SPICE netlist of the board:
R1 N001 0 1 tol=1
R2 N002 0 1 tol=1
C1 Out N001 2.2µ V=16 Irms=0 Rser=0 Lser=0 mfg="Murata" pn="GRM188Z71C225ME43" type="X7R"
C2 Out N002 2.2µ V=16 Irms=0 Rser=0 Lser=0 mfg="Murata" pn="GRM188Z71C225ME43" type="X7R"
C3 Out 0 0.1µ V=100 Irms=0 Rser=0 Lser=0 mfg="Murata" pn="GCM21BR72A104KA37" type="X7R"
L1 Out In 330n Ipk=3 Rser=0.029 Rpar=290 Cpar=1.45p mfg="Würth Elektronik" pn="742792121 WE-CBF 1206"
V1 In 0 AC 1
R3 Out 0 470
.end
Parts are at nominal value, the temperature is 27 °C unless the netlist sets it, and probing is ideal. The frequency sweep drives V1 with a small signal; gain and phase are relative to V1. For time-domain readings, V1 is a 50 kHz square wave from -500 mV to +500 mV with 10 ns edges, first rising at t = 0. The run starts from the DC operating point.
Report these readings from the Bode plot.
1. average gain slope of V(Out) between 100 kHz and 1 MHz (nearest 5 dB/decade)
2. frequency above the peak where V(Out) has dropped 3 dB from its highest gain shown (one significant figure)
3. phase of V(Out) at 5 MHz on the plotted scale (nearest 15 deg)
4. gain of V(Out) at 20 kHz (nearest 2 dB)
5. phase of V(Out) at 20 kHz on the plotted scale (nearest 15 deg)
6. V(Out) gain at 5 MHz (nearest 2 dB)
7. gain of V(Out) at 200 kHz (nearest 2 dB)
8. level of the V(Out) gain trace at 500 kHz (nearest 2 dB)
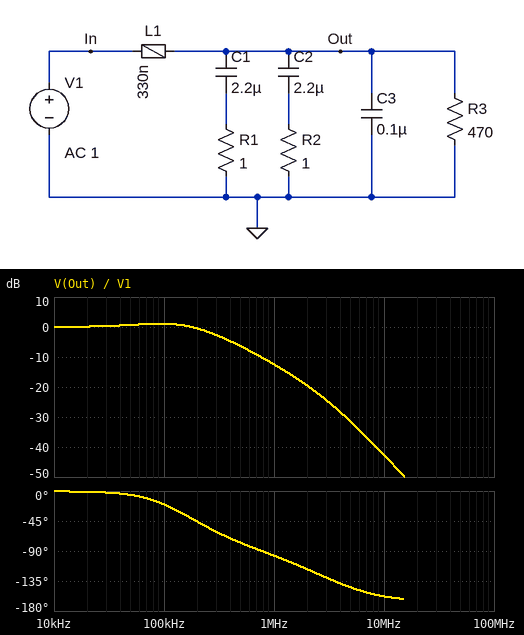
-15 dB/decade
300 kHz
-150 deg
0 dB
0 deg
-32 dB
0 dB
-6 dB
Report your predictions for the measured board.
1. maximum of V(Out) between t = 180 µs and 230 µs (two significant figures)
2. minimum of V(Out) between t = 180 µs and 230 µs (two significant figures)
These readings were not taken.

620 mV
-620 mV
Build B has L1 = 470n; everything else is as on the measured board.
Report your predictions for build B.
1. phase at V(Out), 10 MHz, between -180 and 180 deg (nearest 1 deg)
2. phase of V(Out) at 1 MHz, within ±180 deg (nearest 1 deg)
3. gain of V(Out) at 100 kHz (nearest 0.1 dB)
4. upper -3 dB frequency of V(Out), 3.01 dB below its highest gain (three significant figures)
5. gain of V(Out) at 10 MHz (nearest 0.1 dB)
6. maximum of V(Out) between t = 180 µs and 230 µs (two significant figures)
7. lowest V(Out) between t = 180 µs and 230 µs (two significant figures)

-156 deg
-101 deg
1.4 dB
191 kHz
-45.7 dB
660 mV
-660 mV
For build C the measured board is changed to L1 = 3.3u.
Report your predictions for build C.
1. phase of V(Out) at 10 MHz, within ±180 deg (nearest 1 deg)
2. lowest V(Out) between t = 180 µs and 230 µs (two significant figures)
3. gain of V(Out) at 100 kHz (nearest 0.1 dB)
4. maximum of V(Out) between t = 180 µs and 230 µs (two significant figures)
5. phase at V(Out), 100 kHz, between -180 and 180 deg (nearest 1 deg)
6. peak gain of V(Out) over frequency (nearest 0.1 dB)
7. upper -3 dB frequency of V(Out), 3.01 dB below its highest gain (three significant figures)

-126 deg
-980 mV
-9.4 dB
980 mV
-111 deg
5.9 dB
50.3 kHz
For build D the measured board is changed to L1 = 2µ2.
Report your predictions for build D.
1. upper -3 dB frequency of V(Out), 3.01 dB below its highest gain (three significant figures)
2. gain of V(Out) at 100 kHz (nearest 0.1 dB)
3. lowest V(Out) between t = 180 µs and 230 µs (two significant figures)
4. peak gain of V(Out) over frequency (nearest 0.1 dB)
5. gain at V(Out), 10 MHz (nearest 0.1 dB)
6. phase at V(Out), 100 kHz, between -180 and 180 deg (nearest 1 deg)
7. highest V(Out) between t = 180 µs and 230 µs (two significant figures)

64.0 kHz
-5.5 dB
-1.0 V
4.7 dB
-58.4 dB
-101 deg
1.0 V
